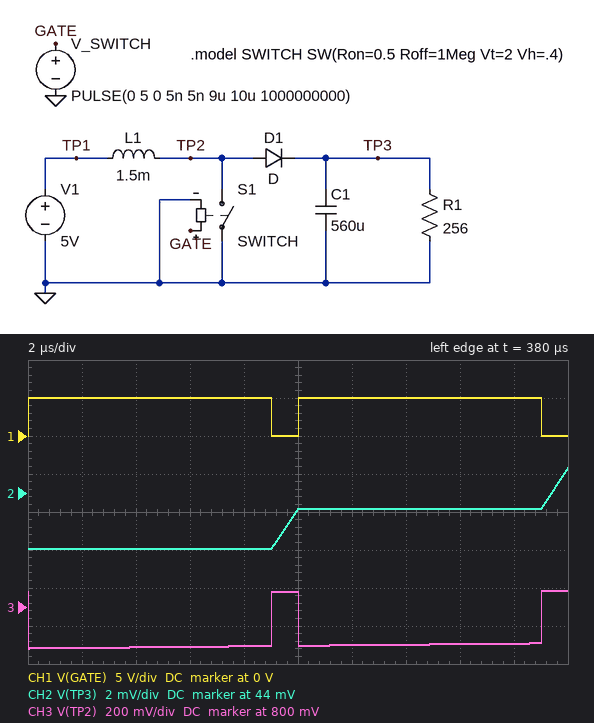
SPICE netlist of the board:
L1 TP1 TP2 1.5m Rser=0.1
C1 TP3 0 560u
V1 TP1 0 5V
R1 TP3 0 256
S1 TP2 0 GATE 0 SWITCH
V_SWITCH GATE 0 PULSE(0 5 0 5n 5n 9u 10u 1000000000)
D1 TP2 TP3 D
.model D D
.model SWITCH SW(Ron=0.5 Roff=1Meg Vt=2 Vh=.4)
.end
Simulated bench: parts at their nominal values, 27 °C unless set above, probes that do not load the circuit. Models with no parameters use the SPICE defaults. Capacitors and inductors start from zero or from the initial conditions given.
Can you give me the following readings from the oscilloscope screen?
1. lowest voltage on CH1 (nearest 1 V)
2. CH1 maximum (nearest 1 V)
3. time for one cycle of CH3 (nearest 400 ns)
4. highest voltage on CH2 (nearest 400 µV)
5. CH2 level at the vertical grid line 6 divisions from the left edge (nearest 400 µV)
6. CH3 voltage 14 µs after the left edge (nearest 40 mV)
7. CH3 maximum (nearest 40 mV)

0 V
5 V
10.0 µs
45.2 mV
43.2 mV
600 mV
880 mV
